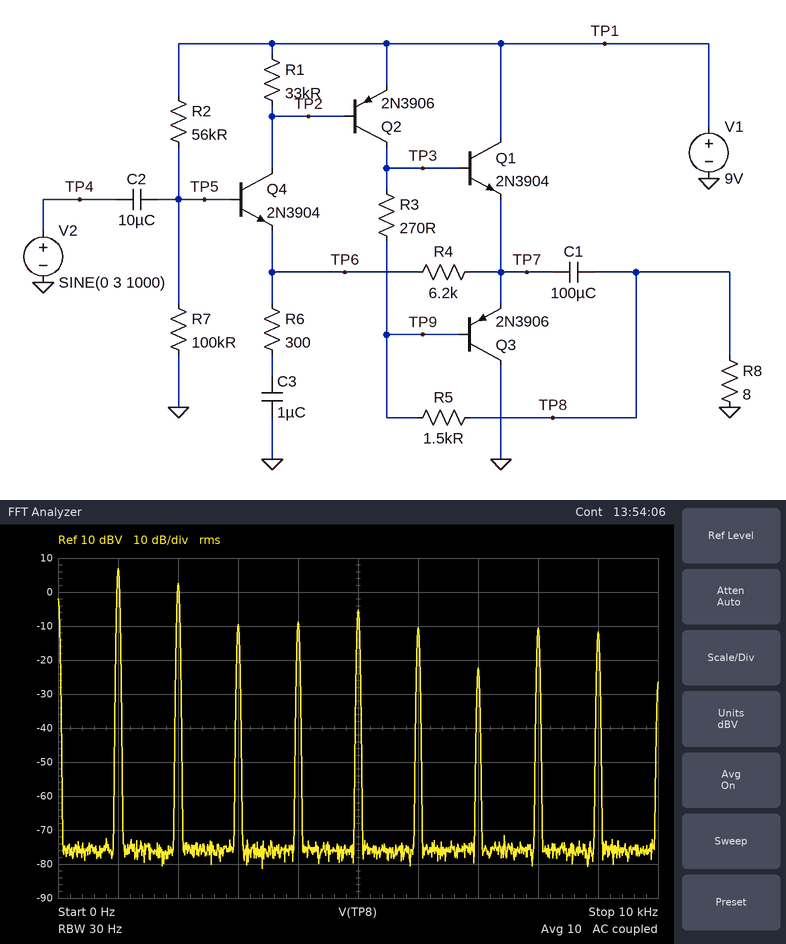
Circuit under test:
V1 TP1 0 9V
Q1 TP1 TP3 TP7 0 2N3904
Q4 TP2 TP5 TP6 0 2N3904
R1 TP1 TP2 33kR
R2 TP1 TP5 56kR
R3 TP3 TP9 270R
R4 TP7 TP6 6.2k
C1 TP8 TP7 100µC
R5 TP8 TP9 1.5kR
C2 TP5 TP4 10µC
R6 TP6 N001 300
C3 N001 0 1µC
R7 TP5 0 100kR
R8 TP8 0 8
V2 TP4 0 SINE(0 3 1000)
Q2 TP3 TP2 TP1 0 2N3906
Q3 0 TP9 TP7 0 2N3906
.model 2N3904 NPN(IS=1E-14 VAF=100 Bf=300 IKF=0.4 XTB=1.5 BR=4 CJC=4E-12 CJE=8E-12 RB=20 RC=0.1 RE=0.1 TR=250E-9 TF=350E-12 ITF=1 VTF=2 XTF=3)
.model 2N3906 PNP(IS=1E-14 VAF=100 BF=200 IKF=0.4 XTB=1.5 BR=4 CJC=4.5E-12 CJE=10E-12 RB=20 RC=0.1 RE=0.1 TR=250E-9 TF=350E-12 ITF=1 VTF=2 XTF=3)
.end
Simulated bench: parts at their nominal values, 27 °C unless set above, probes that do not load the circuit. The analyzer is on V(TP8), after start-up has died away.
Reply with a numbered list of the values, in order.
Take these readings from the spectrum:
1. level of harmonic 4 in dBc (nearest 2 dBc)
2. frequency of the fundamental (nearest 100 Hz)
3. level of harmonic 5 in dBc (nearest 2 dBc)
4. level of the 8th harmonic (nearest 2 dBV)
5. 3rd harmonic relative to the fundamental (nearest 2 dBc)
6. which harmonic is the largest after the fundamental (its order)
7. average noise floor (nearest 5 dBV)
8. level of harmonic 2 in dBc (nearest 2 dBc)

1. -16 dBc
2. 1.0 kHz
3. -12 dBc
4. -10 dBV
5. -16 dBc
6. 2
7. -75 dBV
8. -4 dBc
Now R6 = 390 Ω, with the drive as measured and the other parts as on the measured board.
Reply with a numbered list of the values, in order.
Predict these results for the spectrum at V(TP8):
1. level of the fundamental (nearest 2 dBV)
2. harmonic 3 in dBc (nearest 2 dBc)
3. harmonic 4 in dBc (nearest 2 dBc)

1. 8 dBV
2. -22 dBc
3. -14 dBc
